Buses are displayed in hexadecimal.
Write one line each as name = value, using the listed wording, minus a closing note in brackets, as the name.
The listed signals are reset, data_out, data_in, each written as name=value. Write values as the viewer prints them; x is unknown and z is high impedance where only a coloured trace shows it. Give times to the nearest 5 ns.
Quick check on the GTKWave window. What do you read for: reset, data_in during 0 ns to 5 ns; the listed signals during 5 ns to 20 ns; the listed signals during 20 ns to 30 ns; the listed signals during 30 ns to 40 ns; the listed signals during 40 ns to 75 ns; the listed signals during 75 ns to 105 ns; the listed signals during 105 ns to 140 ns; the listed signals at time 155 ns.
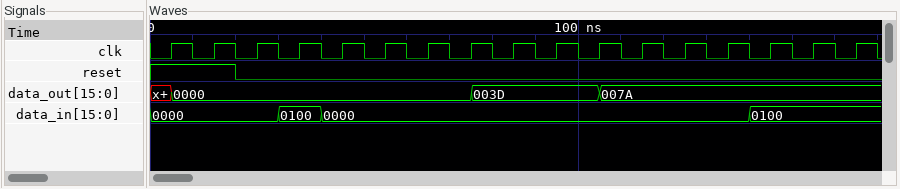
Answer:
reset, data_in during 0 ns to 5 ns = reset=1, data_in=0000
the listed signals during 5 ns to 20 ns = reset=1, data_out=0000, data_in=0000
the listed signals during 20 ns to 30 ns = reset=0, data_out=0000, data_in=0000
the listed signals during 30 ns to 40 ns = reset=0, data_out=0000, data_in=0100
the listed signals during 40 ns to 75 ns = reset=0, data_out=0000, data_in=0000
the listed signals during 75 ns to 105 ns = reset=0, data_out=003D, data_in=0000
the listed signals during 105 ns to 140 ns = reset=0, data_out=007A, data_in=0000
the listed signals at time 155 ns = reset=0, data_out=007A, data_in=0100
